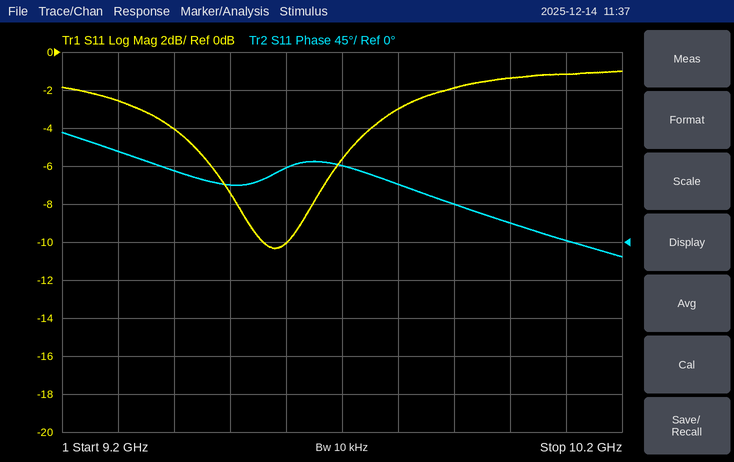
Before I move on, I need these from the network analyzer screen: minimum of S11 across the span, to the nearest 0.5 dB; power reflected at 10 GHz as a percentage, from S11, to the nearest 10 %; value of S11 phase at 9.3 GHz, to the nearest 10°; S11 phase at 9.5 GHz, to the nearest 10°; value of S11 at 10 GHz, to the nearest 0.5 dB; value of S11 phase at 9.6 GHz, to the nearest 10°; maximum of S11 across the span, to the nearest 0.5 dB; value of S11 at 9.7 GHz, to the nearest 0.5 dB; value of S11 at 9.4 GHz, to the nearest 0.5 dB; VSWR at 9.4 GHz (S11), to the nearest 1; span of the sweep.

-10.5 dB
70 %
110°
70°
-1.5 dB
90°
-1.0 dB
-5.5 dB
-4.0 dB
4
1 GHz
